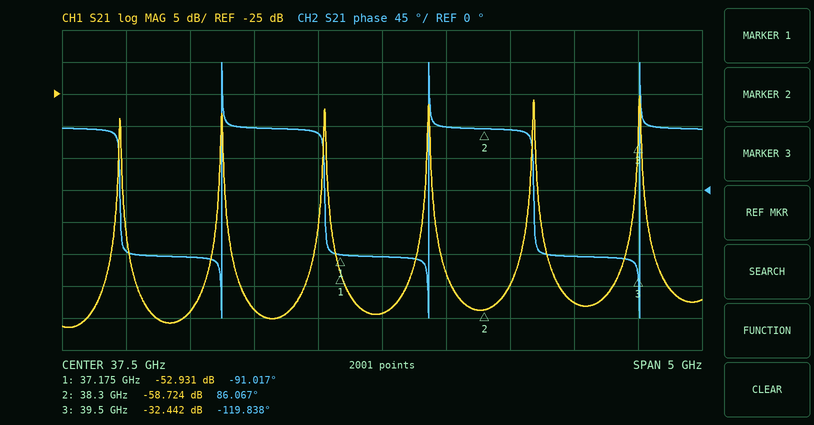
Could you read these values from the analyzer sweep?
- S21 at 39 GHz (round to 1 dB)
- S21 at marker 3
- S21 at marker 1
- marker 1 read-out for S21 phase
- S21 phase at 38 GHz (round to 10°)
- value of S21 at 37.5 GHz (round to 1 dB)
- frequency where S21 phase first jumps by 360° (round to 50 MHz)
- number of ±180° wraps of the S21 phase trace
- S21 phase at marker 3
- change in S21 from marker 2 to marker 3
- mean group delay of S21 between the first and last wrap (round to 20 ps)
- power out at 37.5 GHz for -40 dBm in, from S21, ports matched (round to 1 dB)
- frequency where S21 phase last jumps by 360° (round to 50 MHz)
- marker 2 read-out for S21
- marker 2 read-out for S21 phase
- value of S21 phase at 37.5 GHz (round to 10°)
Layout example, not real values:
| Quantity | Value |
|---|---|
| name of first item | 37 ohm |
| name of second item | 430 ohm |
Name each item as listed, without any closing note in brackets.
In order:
| Quantity | Value |
|---|---|
| S21 at 39 GHz | -58 dB |
| S21 at marker 3 | -32.442 dB |
| S21 at marker 1 | -52.931 dB |
| marker 1 read-out for S21 phase | -91.017° |
| S21 phase at 38 GHz | 90° |
| value of S21 at 37.5 GHz | -59 dB |
| frequency where S21 phase first jumps by 360° | 36.25 GHz |
| number of ±180° wraps of the S21 phase trace | 3 |
| S21 phase at marker 3 | -119.838° |
| change in S21 from marker 2 to marker 3 | 26.282 dB |
| mean group delay of S21 between the first and last wrap | 620 ps |
| power out at 37.5 GHz for -40 dBm in, from S21, ports matched | -99 dBm |
| frequency where S21 phase last jumps by 360° | 39.50 GHz |
| marker 2 read-out for S21 | -58.724 dB |
| marker 2 read-out for S21 phase | 86.067° |
| value of S21 phase at 37.5 GHz | -90° |
